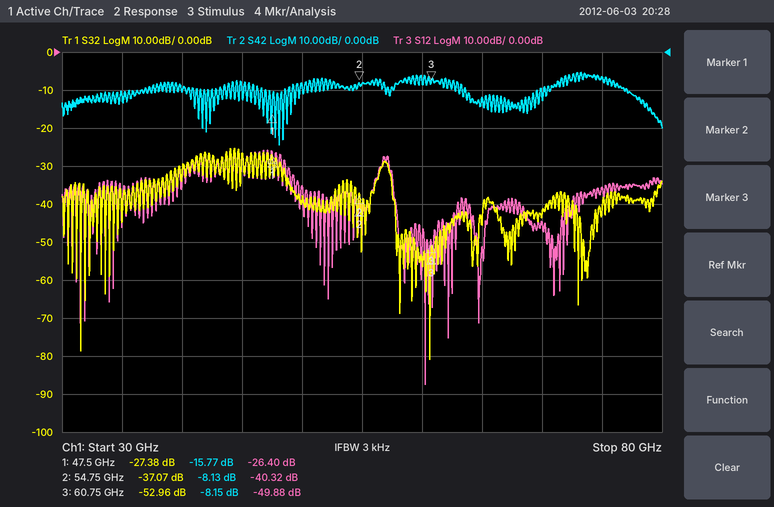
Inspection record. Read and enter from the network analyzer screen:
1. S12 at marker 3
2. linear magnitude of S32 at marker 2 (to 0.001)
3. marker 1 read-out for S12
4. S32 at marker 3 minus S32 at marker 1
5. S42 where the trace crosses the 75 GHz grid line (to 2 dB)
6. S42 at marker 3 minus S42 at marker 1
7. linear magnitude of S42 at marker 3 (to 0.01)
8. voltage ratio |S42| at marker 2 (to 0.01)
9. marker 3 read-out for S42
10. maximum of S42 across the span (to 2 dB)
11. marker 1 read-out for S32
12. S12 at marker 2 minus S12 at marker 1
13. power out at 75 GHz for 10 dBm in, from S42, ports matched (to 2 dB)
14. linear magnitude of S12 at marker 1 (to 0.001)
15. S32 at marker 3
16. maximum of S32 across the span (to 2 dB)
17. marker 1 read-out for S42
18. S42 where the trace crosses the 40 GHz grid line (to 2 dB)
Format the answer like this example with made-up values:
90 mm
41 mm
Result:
-49.88 dB
0.014
-26.40 dB
-25.58 dB
-6 dB
7.62 dB
0.39
0.39
-8.15 dB
-6 dB
-27.38 dB
-13.92 dB
4 dBm
0.048
-52.96 dB
-26 dB
-15.77 dB
-10 dB
